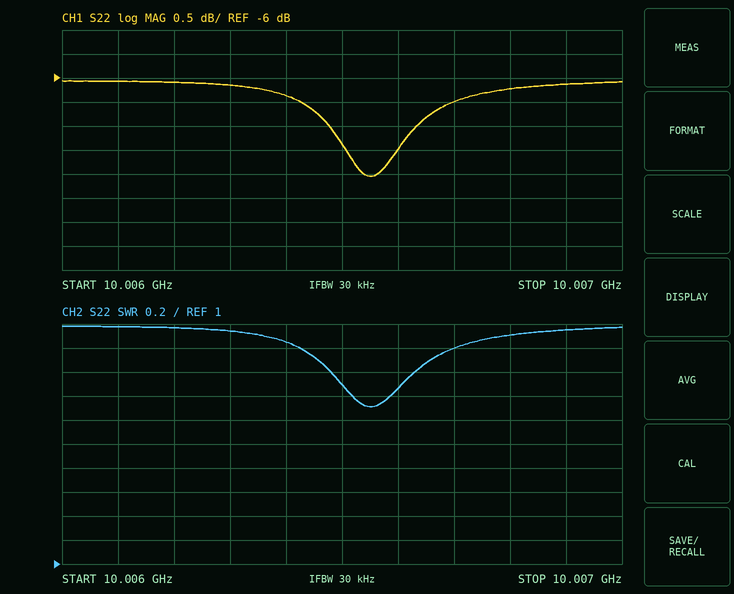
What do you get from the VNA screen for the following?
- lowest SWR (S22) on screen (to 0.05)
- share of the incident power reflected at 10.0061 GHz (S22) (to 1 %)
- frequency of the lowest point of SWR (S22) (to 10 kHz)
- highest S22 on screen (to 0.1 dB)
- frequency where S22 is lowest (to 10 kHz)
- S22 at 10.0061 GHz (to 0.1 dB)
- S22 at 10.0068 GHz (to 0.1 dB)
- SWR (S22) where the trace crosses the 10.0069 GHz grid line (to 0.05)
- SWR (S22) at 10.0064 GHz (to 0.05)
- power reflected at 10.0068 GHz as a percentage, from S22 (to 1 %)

2.30
25 %
10.00655 GHz
-6.1 dB
10.00655 GHz
-6.1 dB
-6.2 dB
2.95
2.85
24 %
